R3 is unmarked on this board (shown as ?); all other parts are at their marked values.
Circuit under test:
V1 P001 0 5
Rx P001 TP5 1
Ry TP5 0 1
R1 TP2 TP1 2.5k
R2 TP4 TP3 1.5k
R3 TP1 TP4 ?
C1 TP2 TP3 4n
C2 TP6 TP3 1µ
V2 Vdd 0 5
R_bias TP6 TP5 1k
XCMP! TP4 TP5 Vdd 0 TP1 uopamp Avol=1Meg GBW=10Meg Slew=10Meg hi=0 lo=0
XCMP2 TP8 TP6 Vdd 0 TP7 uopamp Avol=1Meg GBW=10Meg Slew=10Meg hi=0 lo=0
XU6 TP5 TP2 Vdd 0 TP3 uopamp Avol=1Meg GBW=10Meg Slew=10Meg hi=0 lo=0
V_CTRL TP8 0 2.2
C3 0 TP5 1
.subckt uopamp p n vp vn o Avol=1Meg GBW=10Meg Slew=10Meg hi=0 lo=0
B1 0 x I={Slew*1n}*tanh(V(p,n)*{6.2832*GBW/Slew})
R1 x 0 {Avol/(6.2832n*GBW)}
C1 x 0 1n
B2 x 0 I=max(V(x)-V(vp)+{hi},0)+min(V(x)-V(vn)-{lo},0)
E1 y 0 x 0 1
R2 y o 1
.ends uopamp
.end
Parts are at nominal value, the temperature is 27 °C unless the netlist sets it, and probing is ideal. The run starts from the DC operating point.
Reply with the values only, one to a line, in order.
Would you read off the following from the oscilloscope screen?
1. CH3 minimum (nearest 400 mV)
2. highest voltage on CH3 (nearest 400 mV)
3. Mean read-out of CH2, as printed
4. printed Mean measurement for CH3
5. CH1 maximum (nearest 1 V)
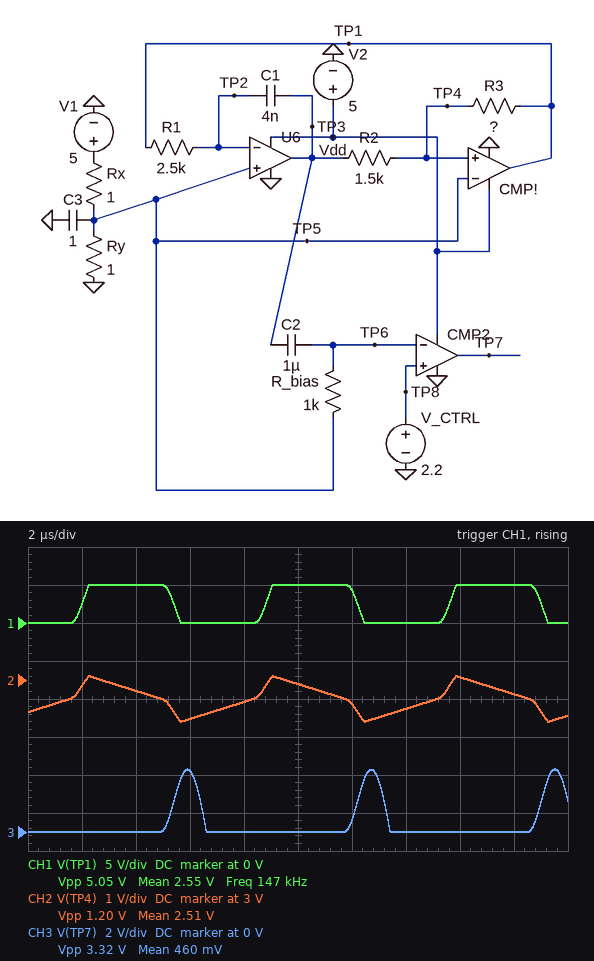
0 V
3.2 V
2.51 V
460 mV
5 V
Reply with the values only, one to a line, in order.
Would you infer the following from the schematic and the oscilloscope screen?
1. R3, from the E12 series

12 kΩ
